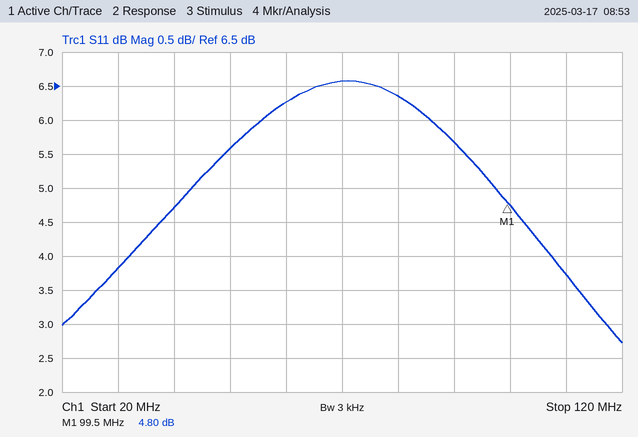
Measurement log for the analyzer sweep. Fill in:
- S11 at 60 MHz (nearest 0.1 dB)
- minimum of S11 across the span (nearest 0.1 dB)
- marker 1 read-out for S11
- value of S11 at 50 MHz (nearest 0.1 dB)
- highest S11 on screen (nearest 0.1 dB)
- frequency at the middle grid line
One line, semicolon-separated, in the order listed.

6.3 dB; 2.7 dB; 4.80 dB; 5.6 dB; 6.6 dB; 70 MHz
